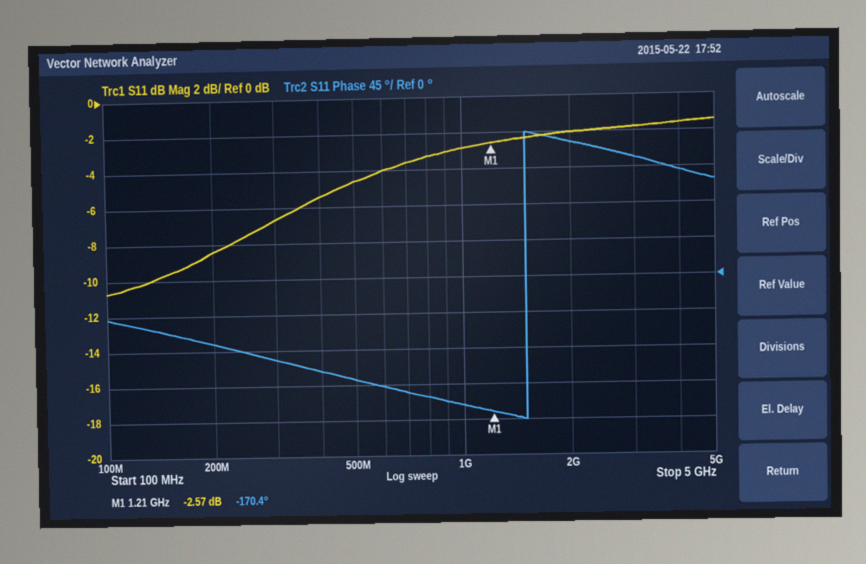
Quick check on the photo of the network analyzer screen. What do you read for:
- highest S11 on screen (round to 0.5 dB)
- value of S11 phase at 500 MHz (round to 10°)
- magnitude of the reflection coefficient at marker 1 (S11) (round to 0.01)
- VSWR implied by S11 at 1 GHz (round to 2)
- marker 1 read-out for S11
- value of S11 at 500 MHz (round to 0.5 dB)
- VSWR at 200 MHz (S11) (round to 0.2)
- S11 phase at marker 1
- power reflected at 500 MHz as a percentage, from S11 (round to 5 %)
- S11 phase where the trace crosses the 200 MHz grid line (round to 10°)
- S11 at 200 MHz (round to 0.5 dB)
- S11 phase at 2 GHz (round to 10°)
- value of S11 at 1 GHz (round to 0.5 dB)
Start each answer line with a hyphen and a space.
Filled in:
- -1.5 dB
- -130°
- 0.74
- 6
- -2.57 dB
- -4.5 dB
- 2.2
- -170.4°
- 35 %
- -80°
- -8.5 dB
- 170°
- -3.0 dB
